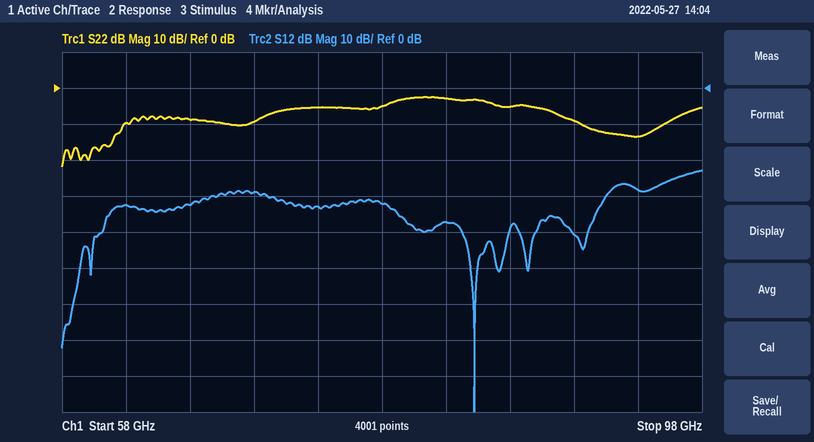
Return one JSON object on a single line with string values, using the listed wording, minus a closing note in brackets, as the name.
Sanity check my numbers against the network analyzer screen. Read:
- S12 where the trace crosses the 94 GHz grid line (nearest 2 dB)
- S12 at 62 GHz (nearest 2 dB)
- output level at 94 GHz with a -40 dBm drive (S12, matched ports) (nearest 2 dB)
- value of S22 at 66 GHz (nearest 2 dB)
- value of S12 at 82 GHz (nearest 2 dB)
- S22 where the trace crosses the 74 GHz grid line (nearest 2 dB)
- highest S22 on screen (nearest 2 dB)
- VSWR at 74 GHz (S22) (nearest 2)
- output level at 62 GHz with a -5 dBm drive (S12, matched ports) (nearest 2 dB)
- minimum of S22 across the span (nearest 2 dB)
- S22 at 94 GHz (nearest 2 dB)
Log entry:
{"S12 where the trace crosses the 94 GHz grid line": "-28 dB", "S12 at 62 GHz": "-32 dB", "output level at 94 GHz with a -40 dBm drive (S12, matched ports)": "-68 dBm", "value of S22 at 66 GHz": "-8 dB", "value of S12 at 82 GHz": "-38 dB", "S22 where the trace crosses the 74 GHz grid line": "-6 dB", "highest S22 on screen": "-2 dB", "VSWR at 74 GHz (S22)": "4", "output level at 62 GHz with a -5 dBm drive (S12, matched ports)": "-38 dBm", "minimum of S22 across the span": "-22 dB", "S22 at 94 GHz": "-14 dB"}
